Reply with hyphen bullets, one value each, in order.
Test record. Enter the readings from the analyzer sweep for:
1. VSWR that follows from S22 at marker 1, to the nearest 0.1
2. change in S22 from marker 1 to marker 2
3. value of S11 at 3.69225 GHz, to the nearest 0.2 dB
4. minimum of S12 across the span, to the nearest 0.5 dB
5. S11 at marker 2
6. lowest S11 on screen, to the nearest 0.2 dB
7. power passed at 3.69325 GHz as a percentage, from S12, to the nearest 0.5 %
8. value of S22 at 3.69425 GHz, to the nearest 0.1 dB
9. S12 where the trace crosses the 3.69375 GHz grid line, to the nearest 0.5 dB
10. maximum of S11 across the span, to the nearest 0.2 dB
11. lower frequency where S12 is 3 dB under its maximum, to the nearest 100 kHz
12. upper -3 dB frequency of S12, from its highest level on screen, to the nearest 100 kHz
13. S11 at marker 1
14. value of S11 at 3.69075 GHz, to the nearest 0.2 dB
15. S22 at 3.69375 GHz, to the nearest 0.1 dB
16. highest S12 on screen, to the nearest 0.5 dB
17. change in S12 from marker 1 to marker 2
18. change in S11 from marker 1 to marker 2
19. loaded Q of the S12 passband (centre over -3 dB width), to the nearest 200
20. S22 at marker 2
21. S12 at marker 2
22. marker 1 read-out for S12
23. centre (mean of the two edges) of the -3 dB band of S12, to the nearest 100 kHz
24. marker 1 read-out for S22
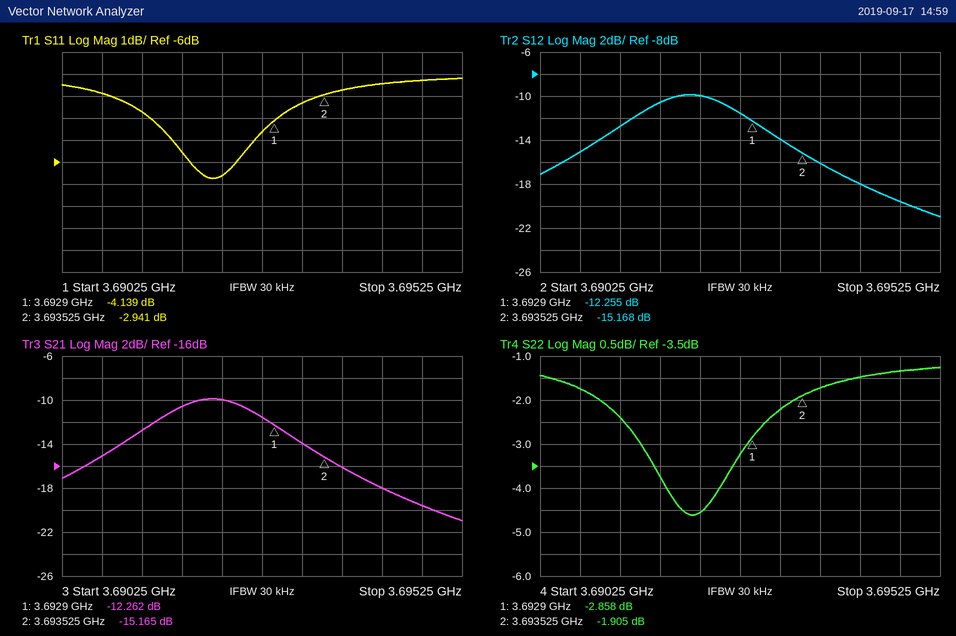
- 6.1
- 0.953 dB
- -6.6 dB
- -21.0 dB
- -2.941 dB
- -6.8 dB
- 4.0 %
- -1.5 dB
- -16.0 dB
- -2.2 dB
- 3.6912 GHz
- 3.6930 GHz
- -4.139 dB
- -2.8 dB
- -1.7 dB
- -10.0 dB
- -2.913 dB
- 1.198 dB
- 2000
- -1.905 dB
- -15.168 dB
- -12.255 dB
- 3.6921 GHz
- -2.858 dB
